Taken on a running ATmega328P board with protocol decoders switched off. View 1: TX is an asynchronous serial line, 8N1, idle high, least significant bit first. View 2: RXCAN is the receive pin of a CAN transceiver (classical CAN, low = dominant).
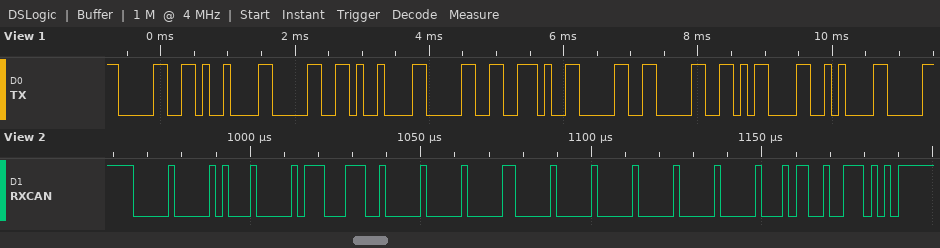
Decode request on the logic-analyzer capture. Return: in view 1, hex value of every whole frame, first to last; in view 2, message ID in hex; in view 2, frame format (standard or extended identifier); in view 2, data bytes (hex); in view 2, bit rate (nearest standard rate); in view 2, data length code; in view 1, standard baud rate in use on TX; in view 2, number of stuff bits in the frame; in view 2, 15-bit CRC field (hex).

30 09 30 09 30 2E 30 30 0D 0A
0x001
standard
1C 72 00 02 00 00 00 00
500 kbit/s
8
9600 baud
12
0x593A
